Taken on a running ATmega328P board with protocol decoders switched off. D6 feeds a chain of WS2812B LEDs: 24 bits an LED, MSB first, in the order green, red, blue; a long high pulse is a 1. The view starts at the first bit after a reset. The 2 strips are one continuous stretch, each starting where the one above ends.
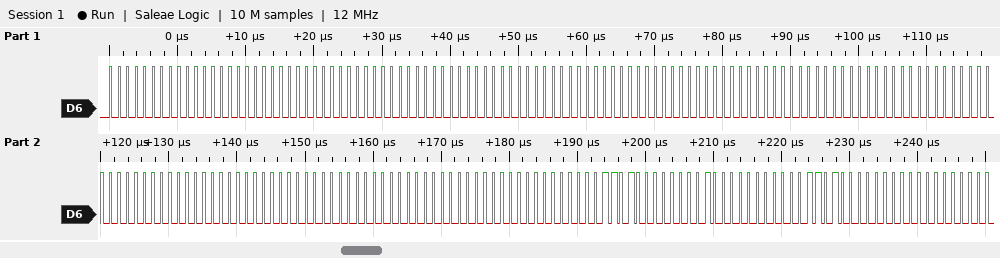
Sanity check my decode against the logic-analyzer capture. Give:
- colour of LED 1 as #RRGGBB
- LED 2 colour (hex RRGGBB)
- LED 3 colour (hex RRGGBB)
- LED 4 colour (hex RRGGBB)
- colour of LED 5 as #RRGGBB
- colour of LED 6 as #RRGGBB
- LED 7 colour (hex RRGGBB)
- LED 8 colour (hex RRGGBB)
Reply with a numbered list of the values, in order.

1. #000000
2. #000000
3. #000000
4. #000000
5. #000000
6. #000000
7. #00001A
8. #00011A
